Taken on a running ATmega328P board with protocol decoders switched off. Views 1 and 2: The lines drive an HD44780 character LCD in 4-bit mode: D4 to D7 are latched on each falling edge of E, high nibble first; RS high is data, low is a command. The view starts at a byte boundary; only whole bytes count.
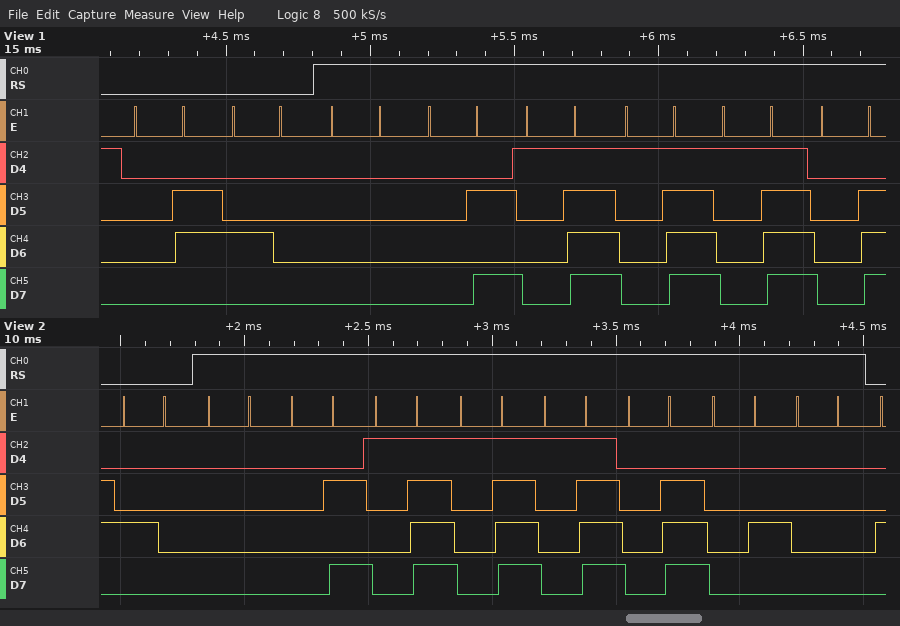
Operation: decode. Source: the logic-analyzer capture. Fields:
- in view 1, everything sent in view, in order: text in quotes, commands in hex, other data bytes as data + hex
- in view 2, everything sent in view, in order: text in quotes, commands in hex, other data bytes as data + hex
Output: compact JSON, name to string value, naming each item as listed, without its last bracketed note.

{"in view 1, everything sent in view, in order: text in quotes, commands in hex, other data bytes as data + hex": "0x06 0x40 data 00 0A 1F 1F 1F 0E", "in view 2, everything sent in view, in order: text in quotes, commands in hex, other data bytes as data + hex": "0x40 data 00 0A 1F 1F 1F 0E 04 00"}
